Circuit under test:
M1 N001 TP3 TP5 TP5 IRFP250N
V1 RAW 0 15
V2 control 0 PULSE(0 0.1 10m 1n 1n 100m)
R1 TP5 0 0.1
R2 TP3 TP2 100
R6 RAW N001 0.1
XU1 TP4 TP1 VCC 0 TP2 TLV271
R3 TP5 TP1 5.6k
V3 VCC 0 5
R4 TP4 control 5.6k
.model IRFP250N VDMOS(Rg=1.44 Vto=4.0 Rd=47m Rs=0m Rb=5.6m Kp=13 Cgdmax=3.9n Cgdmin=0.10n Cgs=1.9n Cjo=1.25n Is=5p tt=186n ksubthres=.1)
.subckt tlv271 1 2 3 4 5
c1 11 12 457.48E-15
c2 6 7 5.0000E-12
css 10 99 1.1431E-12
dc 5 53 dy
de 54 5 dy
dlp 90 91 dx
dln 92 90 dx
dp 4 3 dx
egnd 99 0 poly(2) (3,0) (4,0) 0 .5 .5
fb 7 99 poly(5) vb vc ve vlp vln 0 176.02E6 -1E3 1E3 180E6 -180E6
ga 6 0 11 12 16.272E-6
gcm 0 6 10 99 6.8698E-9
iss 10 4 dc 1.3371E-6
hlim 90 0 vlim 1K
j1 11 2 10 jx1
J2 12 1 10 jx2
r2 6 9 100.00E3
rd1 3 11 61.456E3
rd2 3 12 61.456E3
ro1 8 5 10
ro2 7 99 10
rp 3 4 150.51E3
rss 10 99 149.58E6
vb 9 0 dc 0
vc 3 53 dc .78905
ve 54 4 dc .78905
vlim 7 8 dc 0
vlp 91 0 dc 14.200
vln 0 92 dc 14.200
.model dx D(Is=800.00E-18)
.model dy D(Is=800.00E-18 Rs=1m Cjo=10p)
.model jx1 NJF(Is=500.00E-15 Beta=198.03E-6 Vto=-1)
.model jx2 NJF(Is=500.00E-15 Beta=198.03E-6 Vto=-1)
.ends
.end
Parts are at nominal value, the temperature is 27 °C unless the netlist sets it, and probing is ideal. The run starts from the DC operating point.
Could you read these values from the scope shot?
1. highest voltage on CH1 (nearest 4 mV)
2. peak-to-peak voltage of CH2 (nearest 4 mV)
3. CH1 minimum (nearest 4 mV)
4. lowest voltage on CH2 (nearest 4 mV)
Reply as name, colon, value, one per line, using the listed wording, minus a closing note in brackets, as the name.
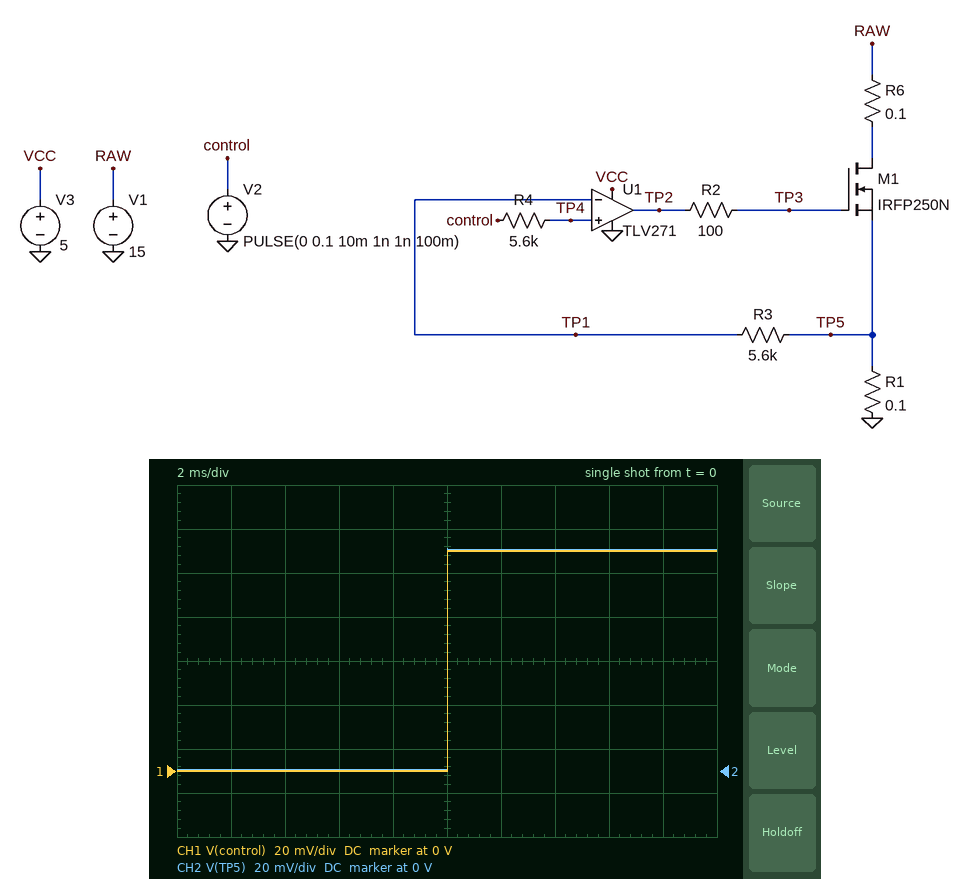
highest voltage on CH1: 100 mV
peak-to-peak voltage of CH2: 100 mV
CH1 minimum: 0 V
lowest voltage on CH2: 0 V
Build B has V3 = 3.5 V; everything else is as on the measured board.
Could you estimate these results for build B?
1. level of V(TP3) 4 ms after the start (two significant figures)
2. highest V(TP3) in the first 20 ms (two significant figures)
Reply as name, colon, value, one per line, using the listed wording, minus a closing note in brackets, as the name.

level of V(TP3) 4 ms after the start: 3.4 V
highest V(TP3) in the first 20 ms: 3.5 V
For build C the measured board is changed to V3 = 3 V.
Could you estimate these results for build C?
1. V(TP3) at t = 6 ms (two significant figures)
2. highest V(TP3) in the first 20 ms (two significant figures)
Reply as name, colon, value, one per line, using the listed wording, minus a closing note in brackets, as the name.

V(TP3) at t = 6 ms: 2.9 V
highest V(TP3) in the first 20 ms: 3.0 V
